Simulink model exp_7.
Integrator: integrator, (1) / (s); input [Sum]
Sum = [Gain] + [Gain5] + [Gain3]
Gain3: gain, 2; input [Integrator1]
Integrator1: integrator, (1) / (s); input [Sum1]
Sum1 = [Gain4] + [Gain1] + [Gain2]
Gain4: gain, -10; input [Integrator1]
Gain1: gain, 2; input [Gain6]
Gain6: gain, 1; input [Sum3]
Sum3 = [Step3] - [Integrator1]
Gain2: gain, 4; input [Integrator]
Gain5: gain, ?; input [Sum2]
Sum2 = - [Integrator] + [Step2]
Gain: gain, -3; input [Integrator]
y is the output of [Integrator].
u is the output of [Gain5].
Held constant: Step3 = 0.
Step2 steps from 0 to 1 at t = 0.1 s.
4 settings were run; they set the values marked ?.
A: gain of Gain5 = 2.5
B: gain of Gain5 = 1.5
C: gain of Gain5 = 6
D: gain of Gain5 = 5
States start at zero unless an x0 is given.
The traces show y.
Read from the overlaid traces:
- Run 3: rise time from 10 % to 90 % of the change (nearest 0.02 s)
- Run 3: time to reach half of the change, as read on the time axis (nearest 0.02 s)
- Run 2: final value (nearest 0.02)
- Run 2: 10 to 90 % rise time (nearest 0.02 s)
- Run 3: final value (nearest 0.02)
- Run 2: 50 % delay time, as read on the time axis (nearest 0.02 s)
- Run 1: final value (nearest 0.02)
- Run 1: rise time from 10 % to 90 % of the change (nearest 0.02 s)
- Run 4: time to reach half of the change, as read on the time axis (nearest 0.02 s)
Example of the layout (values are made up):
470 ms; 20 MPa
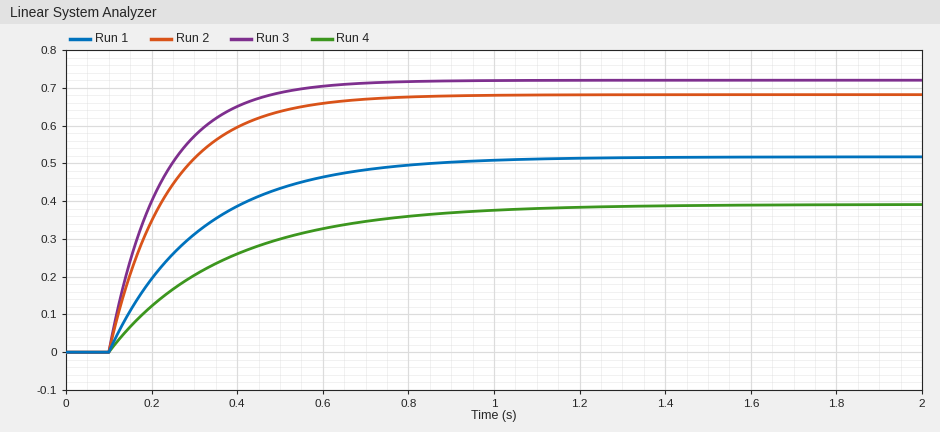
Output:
0.28 s; 0.18 s; 0.68; 0.32 s; 0.72; 0.20 s; 0.52; 0.48 s; 0.28 s
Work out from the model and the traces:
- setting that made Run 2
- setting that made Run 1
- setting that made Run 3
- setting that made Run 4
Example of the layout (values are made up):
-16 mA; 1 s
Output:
D; A; C; B
